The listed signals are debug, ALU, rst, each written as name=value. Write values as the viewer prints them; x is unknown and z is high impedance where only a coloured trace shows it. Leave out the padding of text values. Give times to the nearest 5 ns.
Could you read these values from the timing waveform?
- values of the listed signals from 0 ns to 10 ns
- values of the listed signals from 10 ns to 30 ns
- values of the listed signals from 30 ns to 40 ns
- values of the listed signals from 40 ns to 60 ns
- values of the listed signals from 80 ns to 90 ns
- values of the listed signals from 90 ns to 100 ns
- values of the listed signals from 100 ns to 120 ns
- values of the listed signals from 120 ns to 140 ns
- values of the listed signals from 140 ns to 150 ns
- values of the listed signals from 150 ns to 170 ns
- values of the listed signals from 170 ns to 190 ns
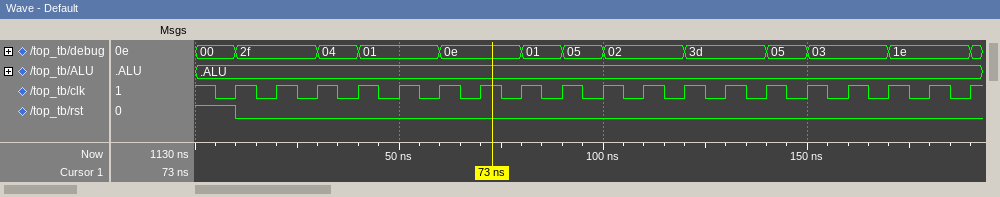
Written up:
debug=00, ALU=ALU, rst=1
debug=2f, ALU=ALU, rst=0
debug=04, ALU=ALU, rst=0
debug=01, ALU=ALU, rst=0
debug=01, ALU=ALU, rst=0
debug=05, ALU=ALU, rst=0
debug=02, ALU=ALU, rst=0
debug=3d, ALU=ALU, rst=0
debug=05, ALU=ALU, rst=0
debug=03, ALU=ALU, rst=0
debug=1e, ALU=ALU, rst=0
